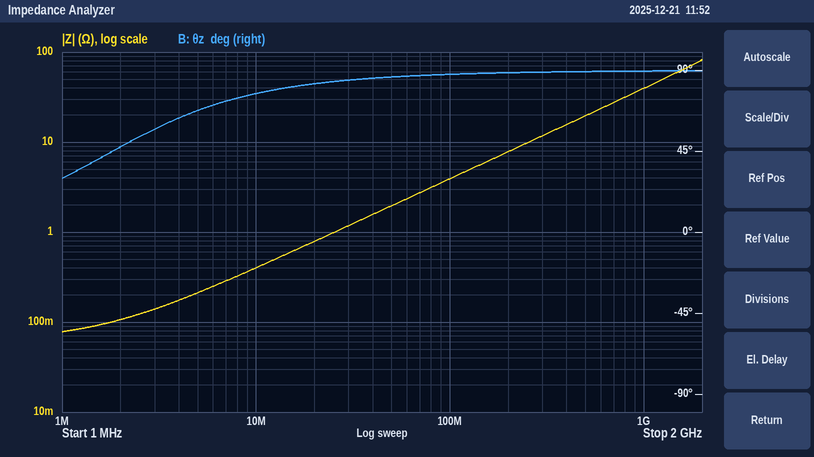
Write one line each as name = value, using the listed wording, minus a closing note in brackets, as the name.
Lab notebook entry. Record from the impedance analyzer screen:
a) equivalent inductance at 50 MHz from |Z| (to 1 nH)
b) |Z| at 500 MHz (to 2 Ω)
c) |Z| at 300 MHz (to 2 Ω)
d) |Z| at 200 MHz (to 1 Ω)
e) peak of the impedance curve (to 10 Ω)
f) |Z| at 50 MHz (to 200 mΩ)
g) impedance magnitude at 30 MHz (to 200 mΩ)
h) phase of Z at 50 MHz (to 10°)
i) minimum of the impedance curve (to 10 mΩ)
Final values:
equivalent inductance at 50 MHz from |Z| = 6 nH
|Z| at 500 MHz = 20 Ω
|Z| at 300 MHz = 12 Ω
|Z| at 200 MHz = 8 Ω
peak of the impedance curve = 80 Ω
|Z| at 50 MHz = 2.0 Ω
impedance magnitude at 30 MHz = 1.2 Ω
phase of Z at 50 MHz = 90°
minimum of the impedance curve = 80 mΩ
